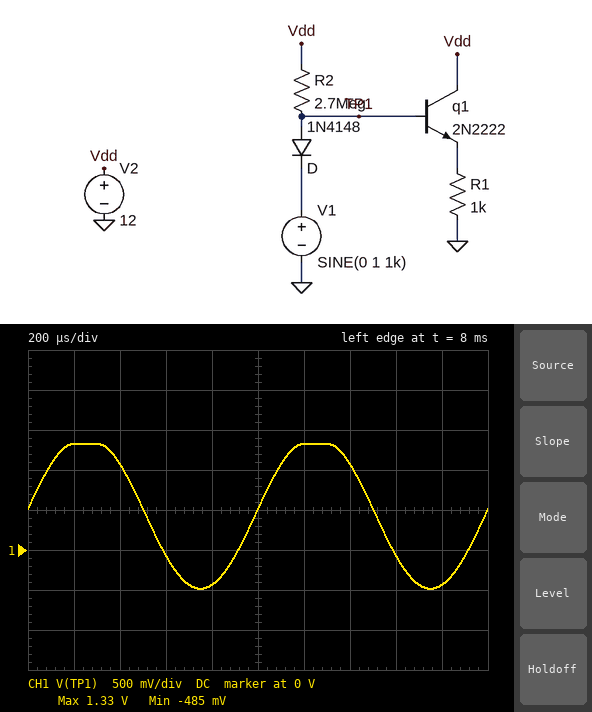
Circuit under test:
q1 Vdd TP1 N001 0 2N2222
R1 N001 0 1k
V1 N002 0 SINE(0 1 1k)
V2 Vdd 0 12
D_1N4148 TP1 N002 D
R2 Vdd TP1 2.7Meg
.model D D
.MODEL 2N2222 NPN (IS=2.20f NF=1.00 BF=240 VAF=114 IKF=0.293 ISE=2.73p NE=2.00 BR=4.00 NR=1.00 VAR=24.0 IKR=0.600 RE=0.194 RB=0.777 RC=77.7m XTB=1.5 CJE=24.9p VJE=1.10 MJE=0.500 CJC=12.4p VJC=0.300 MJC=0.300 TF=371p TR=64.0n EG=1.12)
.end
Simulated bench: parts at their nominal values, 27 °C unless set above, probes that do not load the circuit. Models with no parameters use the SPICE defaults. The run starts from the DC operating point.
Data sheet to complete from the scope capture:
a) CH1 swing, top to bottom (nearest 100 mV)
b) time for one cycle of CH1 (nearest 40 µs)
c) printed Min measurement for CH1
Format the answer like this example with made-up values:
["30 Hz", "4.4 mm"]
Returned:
["1.8 V", "1.00 ms", "-485 mV"]
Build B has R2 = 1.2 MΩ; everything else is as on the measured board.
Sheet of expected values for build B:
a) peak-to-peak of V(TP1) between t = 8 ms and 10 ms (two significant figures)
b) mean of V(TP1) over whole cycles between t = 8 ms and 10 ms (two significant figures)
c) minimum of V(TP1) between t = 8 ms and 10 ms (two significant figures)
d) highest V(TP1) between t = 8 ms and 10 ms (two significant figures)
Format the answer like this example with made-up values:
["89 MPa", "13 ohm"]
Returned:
["2.0 V", "530 mV", "-460 mV", "1.5 V"]
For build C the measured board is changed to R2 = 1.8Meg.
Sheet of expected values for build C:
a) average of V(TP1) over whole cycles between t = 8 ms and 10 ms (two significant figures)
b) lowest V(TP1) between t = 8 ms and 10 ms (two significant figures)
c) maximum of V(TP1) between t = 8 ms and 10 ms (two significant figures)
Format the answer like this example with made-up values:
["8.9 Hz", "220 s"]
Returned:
["510 mV", "-470 mV", "1.5 V"]
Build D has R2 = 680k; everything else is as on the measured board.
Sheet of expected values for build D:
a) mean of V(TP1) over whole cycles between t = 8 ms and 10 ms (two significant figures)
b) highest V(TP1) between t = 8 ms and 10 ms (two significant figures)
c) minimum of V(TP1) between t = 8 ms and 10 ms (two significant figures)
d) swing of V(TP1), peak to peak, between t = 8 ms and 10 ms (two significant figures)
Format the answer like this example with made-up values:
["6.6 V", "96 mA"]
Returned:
["550 mV", "1.5 V", "-450 mV", "2.0 V"]
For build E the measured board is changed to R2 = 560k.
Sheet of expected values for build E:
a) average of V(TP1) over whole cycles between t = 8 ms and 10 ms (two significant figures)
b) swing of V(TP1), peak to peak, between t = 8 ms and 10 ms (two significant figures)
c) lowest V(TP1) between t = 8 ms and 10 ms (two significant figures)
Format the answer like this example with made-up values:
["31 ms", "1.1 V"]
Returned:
["550 mV", "2.0 V", "-440 mV"]
